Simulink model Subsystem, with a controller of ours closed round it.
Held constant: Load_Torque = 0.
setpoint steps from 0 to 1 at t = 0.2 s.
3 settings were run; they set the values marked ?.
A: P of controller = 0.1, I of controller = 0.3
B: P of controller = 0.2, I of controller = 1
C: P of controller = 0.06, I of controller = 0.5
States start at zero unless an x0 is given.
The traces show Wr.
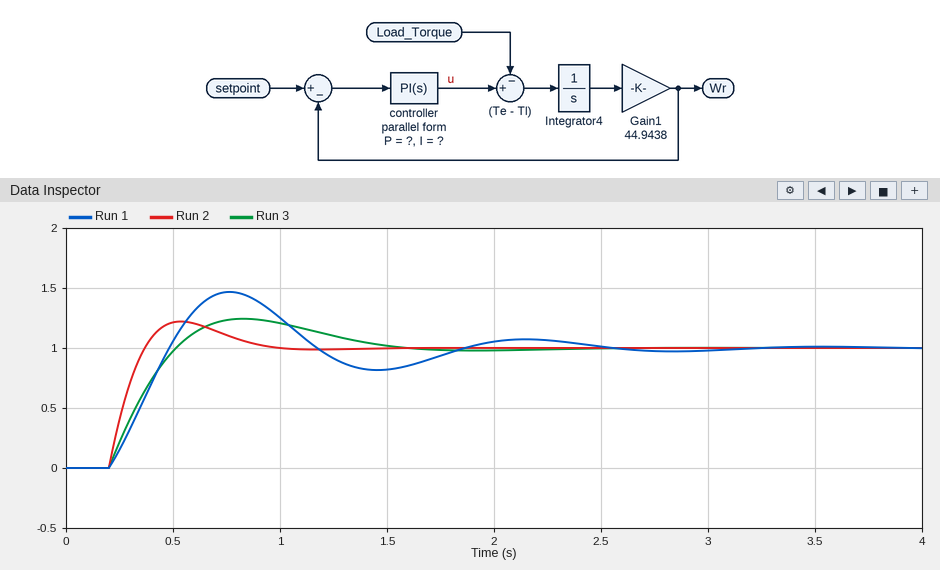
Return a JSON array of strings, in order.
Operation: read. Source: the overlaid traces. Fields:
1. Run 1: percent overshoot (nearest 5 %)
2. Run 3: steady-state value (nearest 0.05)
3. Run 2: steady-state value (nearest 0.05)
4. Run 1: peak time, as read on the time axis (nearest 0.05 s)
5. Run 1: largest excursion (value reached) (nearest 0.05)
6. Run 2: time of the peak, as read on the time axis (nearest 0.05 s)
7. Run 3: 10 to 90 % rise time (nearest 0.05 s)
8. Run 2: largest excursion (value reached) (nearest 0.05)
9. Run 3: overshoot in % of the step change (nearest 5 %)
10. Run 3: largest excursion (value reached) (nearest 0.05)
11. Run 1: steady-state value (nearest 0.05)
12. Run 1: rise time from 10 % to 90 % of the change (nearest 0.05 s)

["45 %", "1.00", "1.00", "0.75 s", "1.45", "0.55 s", "0.25 s", "1.20", "25 %", "1.25", "1.00", "0.20 s"]
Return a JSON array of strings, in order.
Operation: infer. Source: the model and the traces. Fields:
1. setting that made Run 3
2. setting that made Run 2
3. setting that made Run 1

["A", "B", "C"]
